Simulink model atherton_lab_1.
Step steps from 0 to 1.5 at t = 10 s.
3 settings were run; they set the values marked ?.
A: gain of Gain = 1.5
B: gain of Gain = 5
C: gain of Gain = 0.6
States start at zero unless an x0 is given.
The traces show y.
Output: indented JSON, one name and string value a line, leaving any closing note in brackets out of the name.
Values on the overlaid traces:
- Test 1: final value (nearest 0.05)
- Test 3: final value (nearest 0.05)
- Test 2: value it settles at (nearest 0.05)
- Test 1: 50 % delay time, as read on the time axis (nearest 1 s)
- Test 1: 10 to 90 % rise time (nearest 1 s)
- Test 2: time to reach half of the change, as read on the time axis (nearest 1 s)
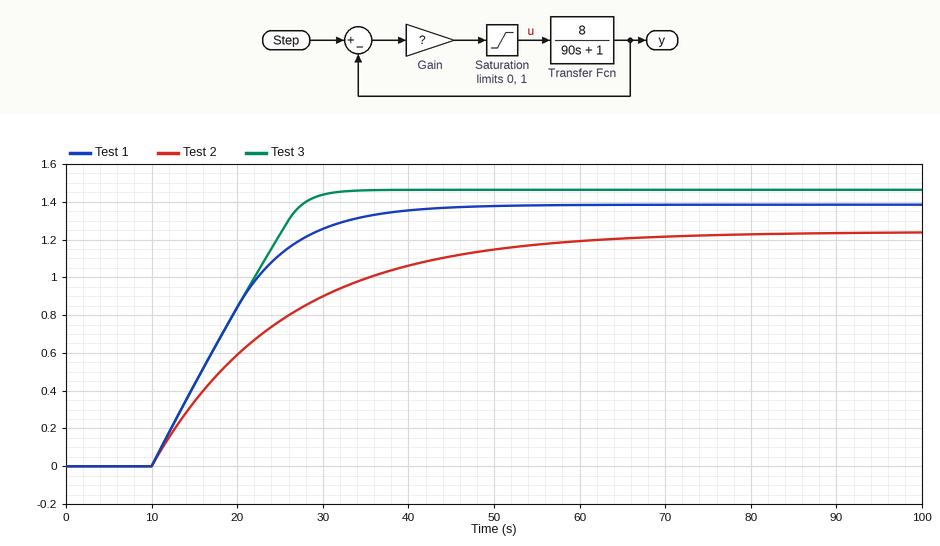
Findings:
{
  "Test 1: final value": "1.40",
  "Test 3: final value": "1.45",
  "Test 2: value it settles at": "1.25",
  "Test 1: 50 % delay time, as read on the time axis": "18 s",
  "Test 1: 10 to 90 % rise time": "18 s",
  "Test 2: time to reach half of the change, as read on the time axis": "21 s"
}
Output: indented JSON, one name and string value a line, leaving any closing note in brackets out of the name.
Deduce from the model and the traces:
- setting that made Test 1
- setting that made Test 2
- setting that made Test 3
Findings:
{
  "setting that made Test 1": "A",
  "setting that made Test 2": "C",
  "setting that made Test 3": "B"
}
